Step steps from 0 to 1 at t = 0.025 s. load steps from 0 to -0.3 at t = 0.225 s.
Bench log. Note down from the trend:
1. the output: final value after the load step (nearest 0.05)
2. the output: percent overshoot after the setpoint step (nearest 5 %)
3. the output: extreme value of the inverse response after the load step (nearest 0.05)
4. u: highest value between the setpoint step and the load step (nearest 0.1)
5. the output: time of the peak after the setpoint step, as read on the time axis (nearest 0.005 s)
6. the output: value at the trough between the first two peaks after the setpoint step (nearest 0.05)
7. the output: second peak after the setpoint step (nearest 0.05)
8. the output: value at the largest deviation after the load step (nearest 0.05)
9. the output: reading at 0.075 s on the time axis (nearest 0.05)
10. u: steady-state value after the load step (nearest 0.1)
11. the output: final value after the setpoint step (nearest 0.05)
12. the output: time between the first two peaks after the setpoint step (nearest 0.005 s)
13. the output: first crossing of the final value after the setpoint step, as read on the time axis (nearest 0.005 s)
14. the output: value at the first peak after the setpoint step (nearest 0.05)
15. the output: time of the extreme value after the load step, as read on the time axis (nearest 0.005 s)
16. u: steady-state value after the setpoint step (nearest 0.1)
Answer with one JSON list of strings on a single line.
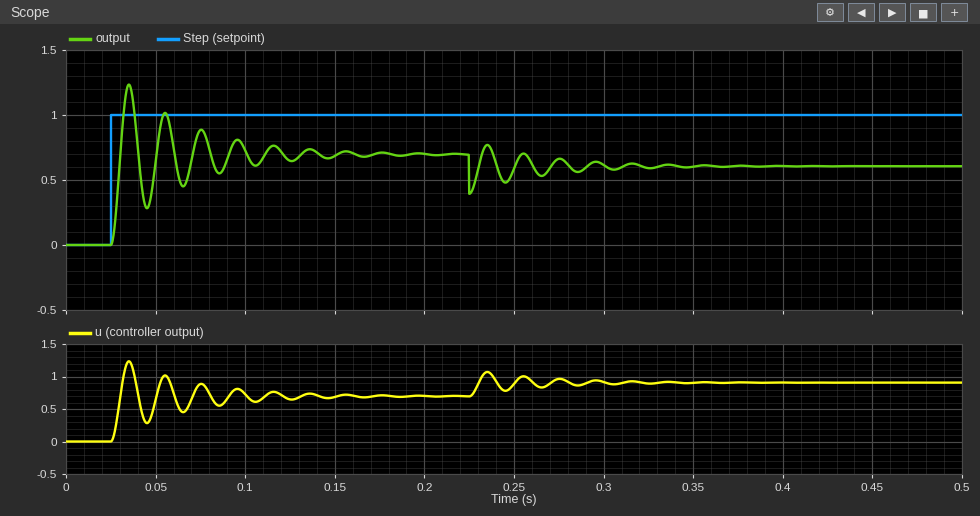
["0.60", "75 %", "0.75", "1.2", "0.035 s", "0.30", "1.00", "0.40", "0.90", "0.9", "0.70", "0.020 s", "0.030 s", "1.25", "0.225 s", "0.7"]
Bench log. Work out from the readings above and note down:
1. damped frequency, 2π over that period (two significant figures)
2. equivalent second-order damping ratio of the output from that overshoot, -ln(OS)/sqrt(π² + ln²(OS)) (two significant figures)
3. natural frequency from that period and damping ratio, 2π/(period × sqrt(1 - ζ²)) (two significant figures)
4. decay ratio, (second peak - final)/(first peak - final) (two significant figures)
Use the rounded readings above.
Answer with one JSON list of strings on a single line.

["310 rad/s", "0.091", "320 rad/s", "0.55"]
